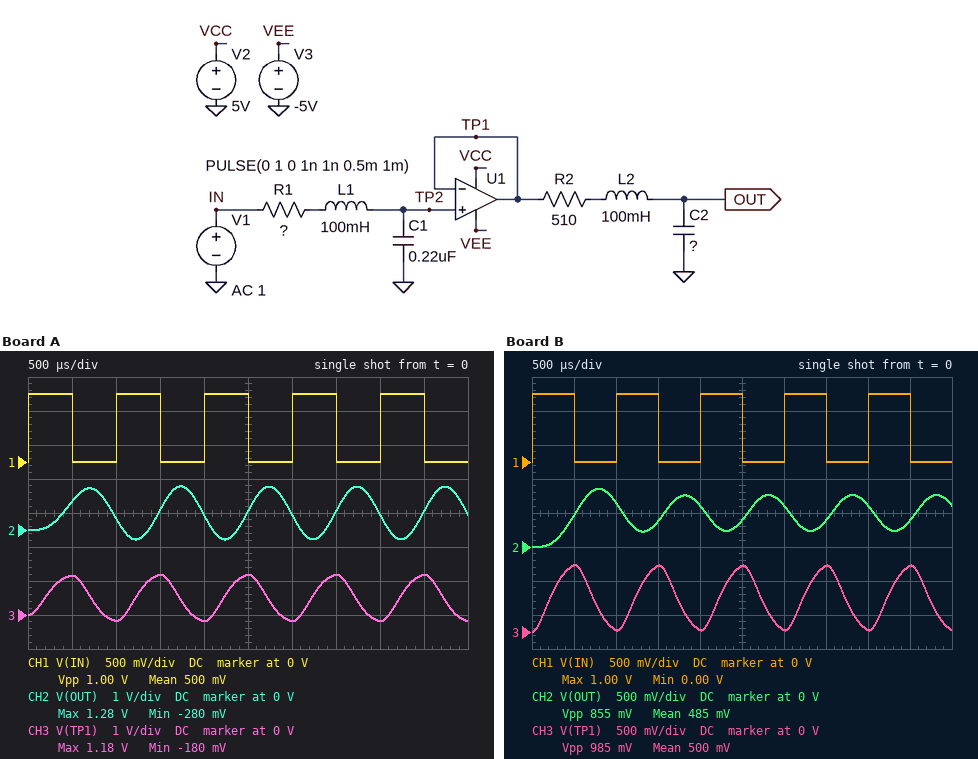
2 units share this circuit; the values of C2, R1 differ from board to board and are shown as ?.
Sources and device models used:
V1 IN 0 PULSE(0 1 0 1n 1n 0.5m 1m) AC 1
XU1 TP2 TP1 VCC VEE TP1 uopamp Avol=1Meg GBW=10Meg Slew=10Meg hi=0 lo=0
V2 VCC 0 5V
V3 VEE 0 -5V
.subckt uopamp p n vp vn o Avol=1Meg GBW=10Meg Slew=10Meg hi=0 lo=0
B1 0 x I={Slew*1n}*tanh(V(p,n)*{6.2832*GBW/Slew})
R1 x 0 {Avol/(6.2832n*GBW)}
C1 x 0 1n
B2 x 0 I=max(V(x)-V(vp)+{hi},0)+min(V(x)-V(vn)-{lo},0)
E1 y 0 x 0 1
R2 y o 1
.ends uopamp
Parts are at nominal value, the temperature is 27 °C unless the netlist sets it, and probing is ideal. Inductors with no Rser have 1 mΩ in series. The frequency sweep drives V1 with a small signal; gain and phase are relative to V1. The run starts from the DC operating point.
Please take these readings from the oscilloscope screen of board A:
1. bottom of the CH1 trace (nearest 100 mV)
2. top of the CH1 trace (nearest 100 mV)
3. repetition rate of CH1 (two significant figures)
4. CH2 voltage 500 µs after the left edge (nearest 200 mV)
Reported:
0 V
1.0 V
1.0 kHz
800 mV
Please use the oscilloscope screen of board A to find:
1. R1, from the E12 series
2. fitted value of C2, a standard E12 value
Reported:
680 Ω
270 nF
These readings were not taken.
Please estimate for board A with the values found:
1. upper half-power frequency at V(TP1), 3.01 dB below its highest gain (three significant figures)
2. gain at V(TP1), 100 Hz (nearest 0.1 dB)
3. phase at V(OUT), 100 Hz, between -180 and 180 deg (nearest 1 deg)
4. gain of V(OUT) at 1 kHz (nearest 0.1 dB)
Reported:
1.25 kHz
0 dB
-10 deg
1.7 dB
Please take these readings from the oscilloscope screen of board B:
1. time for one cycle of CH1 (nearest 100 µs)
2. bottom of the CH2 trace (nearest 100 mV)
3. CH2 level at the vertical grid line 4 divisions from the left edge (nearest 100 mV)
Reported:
1.0 ms
0 V
600 mV
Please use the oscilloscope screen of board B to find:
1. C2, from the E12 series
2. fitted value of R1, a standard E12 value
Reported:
470 nF
1 kΩ
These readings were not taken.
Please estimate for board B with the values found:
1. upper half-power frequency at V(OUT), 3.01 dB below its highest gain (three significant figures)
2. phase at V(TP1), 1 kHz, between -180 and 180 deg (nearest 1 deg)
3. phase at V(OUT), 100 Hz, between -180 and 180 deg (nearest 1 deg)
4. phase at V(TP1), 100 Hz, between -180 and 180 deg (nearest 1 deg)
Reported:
762 Hz
-85 deg
-17 deg
-8 deg
